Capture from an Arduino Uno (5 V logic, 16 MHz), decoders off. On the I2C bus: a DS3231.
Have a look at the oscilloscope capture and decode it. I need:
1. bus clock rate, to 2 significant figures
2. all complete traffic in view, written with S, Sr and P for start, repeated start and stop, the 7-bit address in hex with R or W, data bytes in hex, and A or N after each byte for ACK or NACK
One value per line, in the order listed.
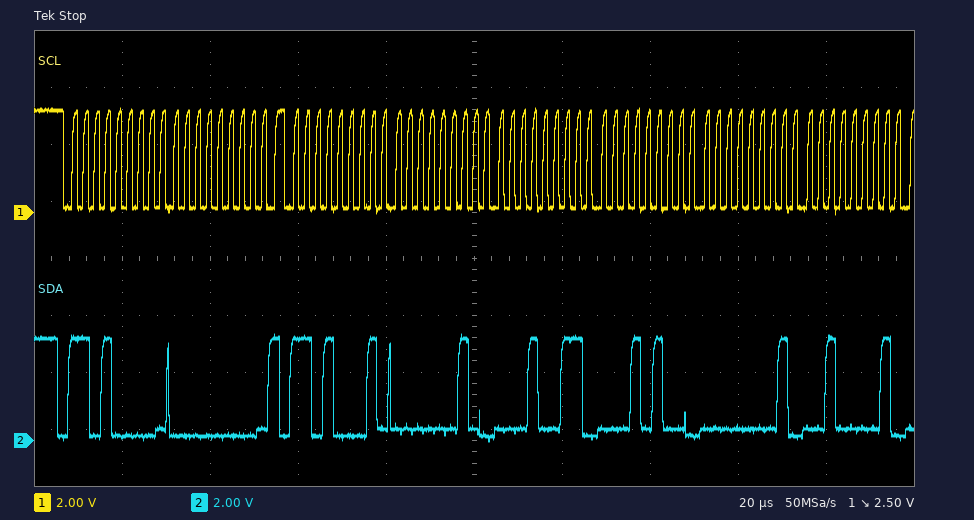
400 kHz
S 68W A 00 A Sr 68R A 02 A 13 A 14 A 01 A 21 A
